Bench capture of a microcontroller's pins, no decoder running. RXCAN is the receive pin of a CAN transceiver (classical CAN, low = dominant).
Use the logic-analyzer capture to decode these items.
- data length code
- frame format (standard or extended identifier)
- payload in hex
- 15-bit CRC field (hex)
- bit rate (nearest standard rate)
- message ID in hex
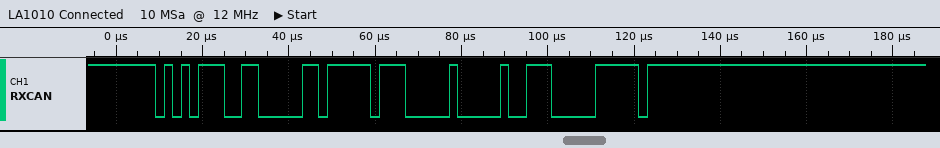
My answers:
2
standard
FF 00
0x0707
500 kbit/s
0x573
